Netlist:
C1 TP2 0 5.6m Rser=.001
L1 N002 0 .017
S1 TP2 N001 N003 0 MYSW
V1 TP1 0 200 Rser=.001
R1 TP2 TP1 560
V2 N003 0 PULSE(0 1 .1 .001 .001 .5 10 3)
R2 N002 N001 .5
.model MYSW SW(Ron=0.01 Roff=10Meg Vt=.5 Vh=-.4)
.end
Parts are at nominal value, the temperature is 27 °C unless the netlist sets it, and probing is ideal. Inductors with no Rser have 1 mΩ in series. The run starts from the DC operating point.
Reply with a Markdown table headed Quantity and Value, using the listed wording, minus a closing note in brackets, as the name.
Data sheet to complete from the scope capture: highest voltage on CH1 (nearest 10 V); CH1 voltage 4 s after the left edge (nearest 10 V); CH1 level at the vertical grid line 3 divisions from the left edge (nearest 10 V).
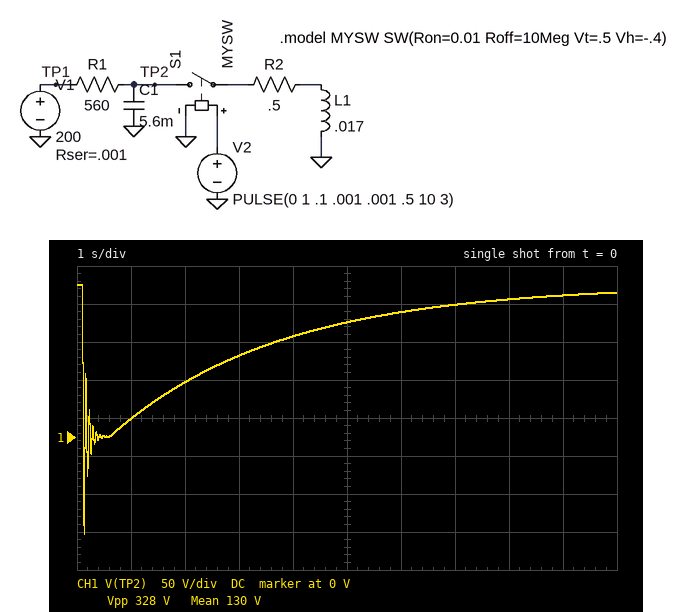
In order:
| Quantity | Value |
|---|---|
| highest voltage on CH1 | 200 V |
| CH1 voltage 4 s after the left edge | 130 V |
| CH1 level at the vertical grid line 3 divisions from the left edge | 110 V |
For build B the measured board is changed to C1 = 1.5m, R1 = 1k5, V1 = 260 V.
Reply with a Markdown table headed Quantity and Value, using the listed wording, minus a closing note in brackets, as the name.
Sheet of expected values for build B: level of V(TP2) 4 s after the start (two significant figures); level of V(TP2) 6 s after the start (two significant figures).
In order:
| Quantity | Value |
|---|---|
| level of V(TP2) 4 s after the start | 200 V |
| level of V(TP2) 6 s after the start | 240 V |
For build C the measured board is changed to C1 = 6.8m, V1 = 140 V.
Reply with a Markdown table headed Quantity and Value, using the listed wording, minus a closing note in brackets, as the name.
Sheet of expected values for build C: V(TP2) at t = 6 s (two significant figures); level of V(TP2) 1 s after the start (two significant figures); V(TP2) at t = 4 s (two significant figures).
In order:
| Quantity | Value |
|---|---|
| V(TP2) at t = 6 s | 110 V |
| level of V(TP2) 1 s after the start | 14 V |
| V(TP2) at t = 4 s | 83 V |
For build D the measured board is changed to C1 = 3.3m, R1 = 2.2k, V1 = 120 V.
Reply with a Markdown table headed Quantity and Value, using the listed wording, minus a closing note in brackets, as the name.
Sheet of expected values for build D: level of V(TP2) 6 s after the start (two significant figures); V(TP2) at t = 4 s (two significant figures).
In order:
| Quantity | Value |
|---|---|
| level of V(TP2) 6 s after the start | 63 V |
| V(TP2) at t = 4 s | 45 V |
